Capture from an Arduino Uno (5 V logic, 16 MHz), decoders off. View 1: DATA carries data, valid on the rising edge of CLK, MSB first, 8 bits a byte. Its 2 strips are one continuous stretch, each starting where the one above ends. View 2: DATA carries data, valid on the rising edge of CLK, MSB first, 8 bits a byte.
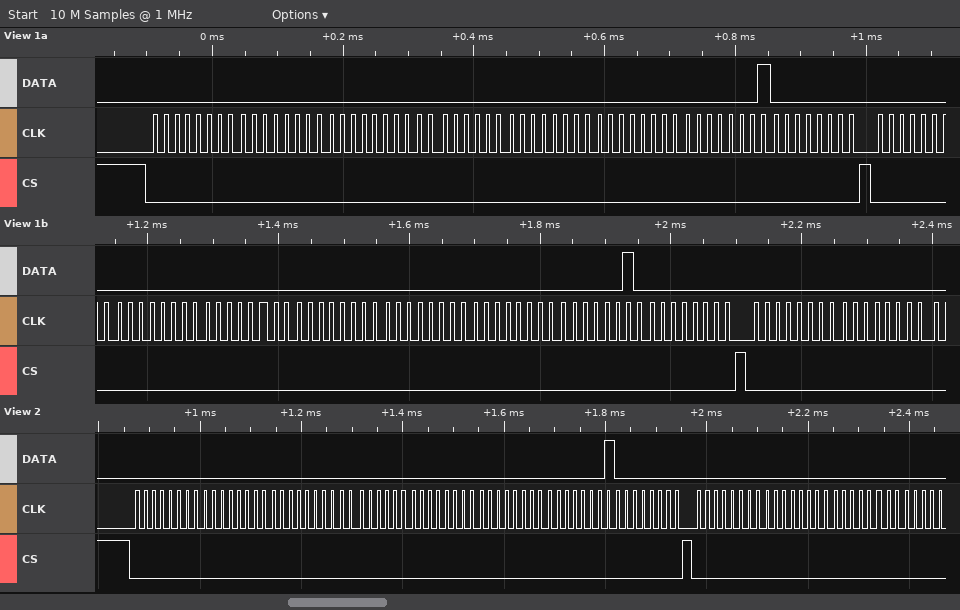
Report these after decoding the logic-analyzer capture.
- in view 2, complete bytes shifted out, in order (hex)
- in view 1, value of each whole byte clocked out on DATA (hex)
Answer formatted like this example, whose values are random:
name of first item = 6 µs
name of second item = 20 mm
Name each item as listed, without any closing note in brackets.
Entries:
in view 2, complete bytes shifted out, in order = 00 00 00 00 00 00 01 00 00 00 00
in view 1, value of each whole byte clocked out on DATA = 00 00 00 00 00 00 01 00 00 00 00 00 00 00 02 00 00 00
